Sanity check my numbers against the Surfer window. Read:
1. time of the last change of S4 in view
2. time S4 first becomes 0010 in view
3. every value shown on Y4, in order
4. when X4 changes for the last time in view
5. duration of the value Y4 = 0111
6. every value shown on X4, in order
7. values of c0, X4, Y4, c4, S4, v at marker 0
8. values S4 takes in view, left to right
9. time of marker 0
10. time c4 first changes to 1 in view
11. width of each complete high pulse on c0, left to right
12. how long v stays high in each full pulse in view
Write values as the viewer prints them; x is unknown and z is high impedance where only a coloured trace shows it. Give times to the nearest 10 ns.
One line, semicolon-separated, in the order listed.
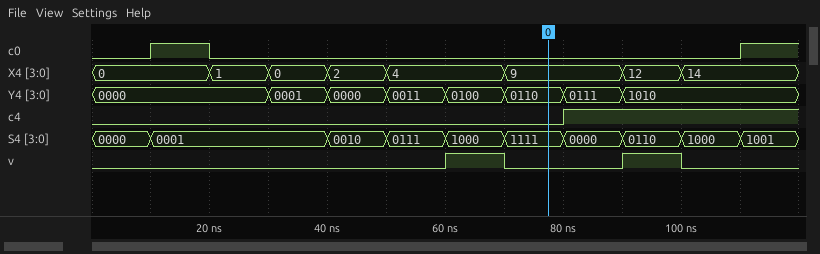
110 ns; 40 ns; 0000, 0001, 0000, 0011, 0100, 0110, 0111, 1010; 100 ns; 10 ns; 0, 1, 0, 2, 4, 9, 12, 14; c0=0, X4=9, Y4=0110, c4=0, S4=1111, v=0; 0000, 0001, 0010, 0111, 1000, 1111, 0000, 0110, 1000, 1001; 80 ns; 80 ns; 10 ns; 10 ns, 10 ns
